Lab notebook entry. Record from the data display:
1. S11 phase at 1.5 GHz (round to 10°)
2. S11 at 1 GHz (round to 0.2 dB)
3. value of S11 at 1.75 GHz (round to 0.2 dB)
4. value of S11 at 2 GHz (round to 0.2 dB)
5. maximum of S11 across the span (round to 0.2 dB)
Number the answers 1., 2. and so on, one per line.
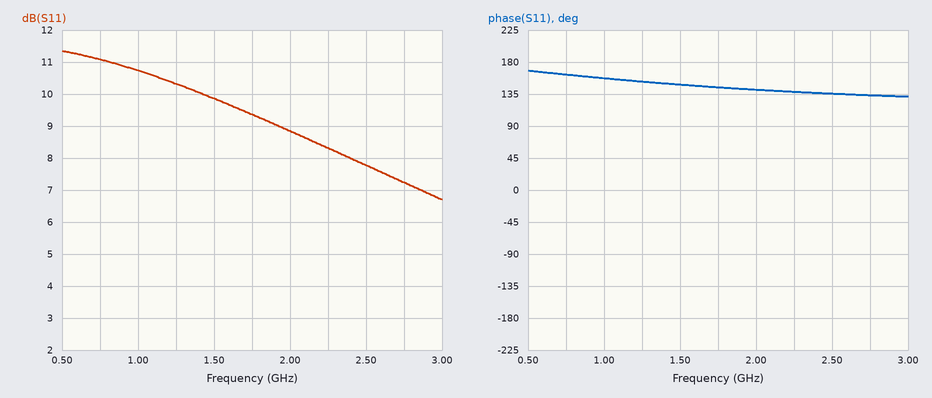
1. 150°
2. 10.8 dB
3. 9.4 dB
4. 8.8 dB
5. 11.4 dB
